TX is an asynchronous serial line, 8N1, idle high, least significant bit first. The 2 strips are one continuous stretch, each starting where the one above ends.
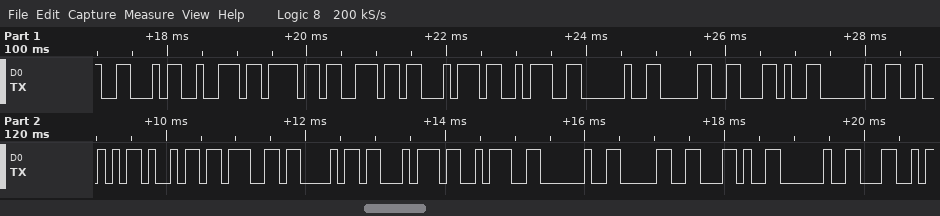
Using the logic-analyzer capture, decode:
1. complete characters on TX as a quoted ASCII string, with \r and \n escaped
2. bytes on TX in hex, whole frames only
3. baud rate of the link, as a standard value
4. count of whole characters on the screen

"Front: 0, Right: 0, L"
0x46 0x72 0x6F 0x6E 0x74 0x3A 0x20 0x30 0x2C 0x20 0x52 0x69 0x67 0x68 0x74 0x3A 0x20 0x30 0x2C 0x20 0x4C
9600 baud
21
